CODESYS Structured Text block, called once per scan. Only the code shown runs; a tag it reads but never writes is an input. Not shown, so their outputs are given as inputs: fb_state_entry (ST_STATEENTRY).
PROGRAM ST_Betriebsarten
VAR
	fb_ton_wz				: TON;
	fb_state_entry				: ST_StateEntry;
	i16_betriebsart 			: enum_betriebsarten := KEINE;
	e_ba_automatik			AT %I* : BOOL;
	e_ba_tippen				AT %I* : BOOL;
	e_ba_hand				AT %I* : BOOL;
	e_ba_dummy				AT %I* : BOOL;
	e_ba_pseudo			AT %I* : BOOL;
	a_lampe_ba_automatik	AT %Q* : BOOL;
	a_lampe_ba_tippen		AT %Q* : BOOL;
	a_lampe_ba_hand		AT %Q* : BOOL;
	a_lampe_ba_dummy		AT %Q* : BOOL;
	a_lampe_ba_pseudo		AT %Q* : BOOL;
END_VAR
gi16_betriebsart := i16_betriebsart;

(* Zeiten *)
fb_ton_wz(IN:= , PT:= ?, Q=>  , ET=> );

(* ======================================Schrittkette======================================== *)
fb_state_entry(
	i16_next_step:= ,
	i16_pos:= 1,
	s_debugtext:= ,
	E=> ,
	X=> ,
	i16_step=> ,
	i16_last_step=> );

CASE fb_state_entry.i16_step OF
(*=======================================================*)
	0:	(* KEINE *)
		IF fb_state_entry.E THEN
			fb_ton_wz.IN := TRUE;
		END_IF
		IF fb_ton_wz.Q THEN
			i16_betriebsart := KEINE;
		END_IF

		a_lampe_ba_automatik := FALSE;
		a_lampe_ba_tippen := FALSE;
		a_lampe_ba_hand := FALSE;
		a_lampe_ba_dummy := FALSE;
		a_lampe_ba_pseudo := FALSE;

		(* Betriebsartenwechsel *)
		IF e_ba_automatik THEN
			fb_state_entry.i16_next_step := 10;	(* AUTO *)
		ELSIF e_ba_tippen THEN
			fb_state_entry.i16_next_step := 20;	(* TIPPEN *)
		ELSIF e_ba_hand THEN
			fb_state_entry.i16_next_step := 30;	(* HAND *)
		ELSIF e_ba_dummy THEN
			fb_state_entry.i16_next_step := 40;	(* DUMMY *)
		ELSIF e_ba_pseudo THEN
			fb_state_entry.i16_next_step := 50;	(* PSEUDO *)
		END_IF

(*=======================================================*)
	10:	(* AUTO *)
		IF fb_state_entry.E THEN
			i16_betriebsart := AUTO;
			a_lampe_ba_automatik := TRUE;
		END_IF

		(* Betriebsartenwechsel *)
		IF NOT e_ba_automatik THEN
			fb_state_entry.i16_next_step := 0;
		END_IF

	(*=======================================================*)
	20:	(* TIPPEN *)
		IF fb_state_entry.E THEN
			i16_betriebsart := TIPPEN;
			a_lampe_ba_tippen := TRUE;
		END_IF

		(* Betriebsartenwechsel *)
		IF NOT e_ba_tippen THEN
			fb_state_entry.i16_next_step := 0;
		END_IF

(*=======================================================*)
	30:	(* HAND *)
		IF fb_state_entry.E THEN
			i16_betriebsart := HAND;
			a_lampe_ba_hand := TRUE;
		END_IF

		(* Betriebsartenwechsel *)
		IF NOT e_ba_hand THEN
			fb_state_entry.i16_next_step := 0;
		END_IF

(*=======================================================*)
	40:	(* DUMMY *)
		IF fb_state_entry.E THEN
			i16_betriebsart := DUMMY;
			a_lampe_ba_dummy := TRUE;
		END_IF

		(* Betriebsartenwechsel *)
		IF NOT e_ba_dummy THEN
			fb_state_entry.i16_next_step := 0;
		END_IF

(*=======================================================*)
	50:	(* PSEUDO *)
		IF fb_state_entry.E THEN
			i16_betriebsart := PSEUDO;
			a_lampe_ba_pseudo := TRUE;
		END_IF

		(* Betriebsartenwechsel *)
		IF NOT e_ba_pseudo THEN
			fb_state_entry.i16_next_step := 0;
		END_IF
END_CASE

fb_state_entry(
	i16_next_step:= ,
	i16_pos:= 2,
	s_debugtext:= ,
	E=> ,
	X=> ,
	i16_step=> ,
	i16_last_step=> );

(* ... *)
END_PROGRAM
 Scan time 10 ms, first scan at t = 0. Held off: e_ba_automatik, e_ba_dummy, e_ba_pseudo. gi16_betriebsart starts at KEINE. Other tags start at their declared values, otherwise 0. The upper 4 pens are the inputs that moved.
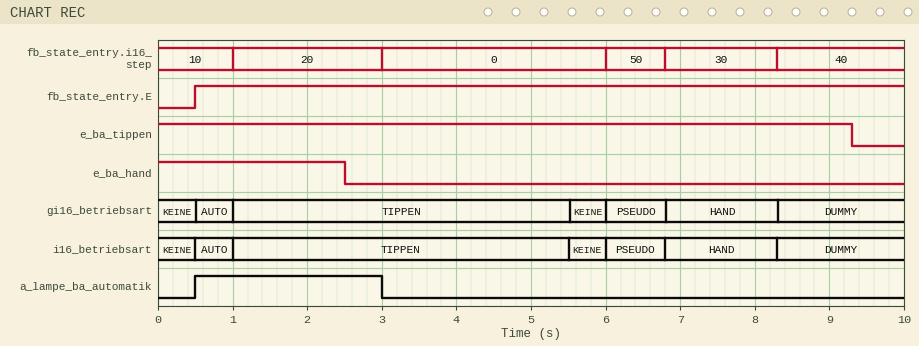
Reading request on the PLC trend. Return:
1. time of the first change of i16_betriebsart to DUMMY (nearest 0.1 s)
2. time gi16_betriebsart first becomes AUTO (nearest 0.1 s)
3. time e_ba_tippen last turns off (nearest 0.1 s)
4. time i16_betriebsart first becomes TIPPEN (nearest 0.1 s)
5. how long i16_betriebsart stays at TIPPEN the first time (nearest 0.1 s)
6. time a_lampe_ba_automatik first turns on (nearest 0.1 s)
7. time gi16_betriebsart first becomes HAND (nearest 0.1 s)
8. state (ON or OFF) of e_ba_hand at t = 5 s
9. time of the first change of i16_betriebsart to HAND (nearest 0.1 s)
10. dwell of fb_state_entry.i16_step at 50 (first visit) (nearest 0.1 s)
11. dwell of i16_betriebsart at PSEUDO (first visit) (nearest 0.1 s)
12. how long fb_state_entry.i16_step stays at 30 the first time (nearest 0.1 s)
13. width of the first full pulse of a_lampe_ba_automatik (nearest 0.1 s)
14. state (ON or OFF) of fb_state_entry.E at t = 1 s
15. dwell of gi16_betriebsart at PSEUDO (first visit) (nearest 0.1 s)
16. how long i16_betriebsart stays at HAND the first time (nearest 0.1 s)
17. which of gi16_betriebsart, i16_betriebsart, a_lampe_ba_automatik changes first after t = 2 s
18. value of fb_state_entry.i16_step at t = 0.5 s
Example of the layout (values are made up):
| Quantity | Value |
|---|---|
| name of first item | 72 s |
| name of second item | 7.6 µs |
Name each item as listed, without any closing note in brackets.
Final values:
| Quantity | Value |
|---|---|
| time of the first change of i16_betriebsart to DUMMY | 8.3 s |
| time gi16_betriebsart first becomes AUTO | 0.5 s |
| time e_ba_tippen last turns off | 9.3 s |
| time i16_betriebsart first becomes TIPPEN | 1.0 s |
| how long i16_betriebsart stays at TIPPEN the first time | 4.5 s |
| time a_lampe_ba_automatik first turns on | 0.5 s |
| time gi16_betriebsart first becomes HAND | 6.8 s |
| state (ON or OFF) of e_ba_hand at t = 5 s | OFF |
| time of the first change of i16_betriebsart to HAND | 6.8 s |
| dwell of fb_state_entry.i16_step at 50 (first visit) | 0.8 s |
| dwell of i16_betriebsart at PSEUDO (first visit) | 0.8 s |
| how long fb_state_entry.i16_step stays at 30 the first time | 1.5 s |
| width of the first full pulse of a_lampe_ba_automatik | 2.5 s |
| state (ON or OFF) of fb_state_entry.E at t = 1 s | ON |
| dwell of gi16_betriebsart at PSEUDO (first visit) | 0.8 s |
| how long i16_betriebsart stays at HAND the first time | 1.5 s |
| which of gi16_betriebsart, i16_betriebsart, a_lampe_ba_automatik changes first after t = 2 s | a_lampe_ba_automatik |
| value of fb_state_entry.i16_step at t = 0.5 s | 10 |
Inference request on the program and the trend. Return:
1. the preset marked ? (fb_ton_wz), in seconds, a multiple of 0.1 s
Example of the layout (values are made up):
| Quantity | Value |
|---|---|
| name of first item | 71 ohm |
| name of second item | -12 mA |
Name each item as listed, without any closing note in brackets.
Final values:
| Quantity | Value |
|---|---|
| the preset marked ? (fb_ton_wz), in seconds, a multiple of 0.1 s | 2.5 s |
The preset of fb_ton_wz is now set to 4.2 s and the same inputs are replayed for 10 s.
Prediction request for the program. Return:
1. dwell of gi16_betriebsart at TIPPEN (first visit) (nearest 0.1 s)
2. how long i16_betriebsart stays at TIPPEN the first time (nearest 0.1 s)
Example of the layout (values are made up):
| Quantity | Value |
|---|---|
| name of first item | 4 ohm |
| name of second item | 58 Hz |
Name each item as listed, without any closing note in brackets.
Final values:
| Quantity | Value |
|---|---|
| dwell of gi16_betriebsart at TIPPEN (first visit) | 5.0 s |
| how long i16_betriebsart stays at TIPPEN the first time | 5.0 s |
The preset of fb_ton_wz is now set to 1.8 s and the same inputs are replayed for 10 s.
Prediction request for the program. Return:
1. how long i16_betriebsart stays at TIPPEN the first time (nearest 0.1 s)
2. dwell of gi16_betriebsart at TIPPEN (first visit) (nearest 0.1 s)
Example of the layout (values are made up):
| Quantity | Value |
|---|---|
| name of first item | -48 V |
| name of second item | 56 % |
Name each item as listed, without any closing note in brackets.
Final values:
| Quantity | Value |
|---|---|
| how long i16_betriebsart stays at TIPPEN the first time | 3.8 s |
| dwell of gi16_betriebsart at TIPPEN (first visit) | 3.8 s |
